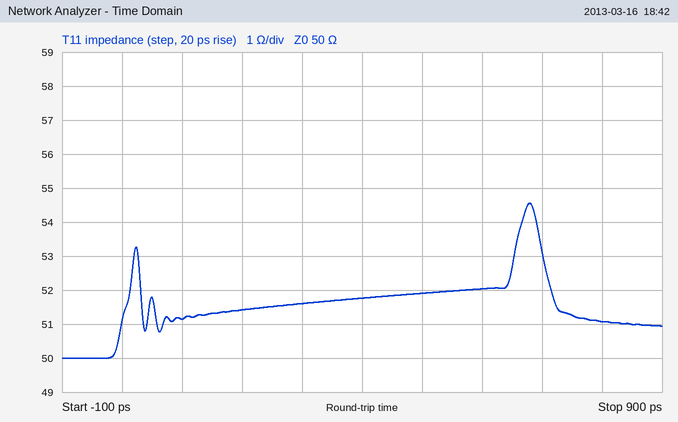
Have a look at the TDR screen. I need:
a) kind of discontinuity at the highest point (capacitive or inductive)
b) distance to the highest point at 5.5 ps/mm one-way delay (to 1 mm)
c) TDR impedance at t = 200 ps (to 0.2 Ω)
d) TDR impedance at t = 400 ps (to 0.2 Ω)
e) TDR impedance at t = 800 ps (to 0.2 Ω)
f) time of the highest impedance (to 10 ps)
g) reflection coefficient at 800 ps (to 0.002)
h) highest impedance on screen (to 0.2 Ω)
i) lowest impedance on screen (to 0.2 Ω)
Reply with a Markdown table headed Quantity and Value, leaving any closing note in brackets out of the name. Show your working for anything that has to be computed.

| Quantity | Value |
|---|---|
| kind of discontinuity at the highest point | inductive |
| distance to the highest point at 5.5 ps/mm one-way delay | 680 ps / 2 / 5.5 ps/mm ≈ 62 mm |
| TDR impedance at t = 200 ps | 51.4 Ω |
| TDR impedance at t = 400 ps | 51.8 Ω |
| TDR impedance at t = 800 ps | 51.0 Ω |
| time of the highest impedance | 680 ps |
| reflection coefficient at 800 ps | (51 − 50)/(51 + 50) ≈ +0.010 |
| highest impedance on screen | 54.6 Ω |
| lowest impedance on screen | 50.0 Ω |
